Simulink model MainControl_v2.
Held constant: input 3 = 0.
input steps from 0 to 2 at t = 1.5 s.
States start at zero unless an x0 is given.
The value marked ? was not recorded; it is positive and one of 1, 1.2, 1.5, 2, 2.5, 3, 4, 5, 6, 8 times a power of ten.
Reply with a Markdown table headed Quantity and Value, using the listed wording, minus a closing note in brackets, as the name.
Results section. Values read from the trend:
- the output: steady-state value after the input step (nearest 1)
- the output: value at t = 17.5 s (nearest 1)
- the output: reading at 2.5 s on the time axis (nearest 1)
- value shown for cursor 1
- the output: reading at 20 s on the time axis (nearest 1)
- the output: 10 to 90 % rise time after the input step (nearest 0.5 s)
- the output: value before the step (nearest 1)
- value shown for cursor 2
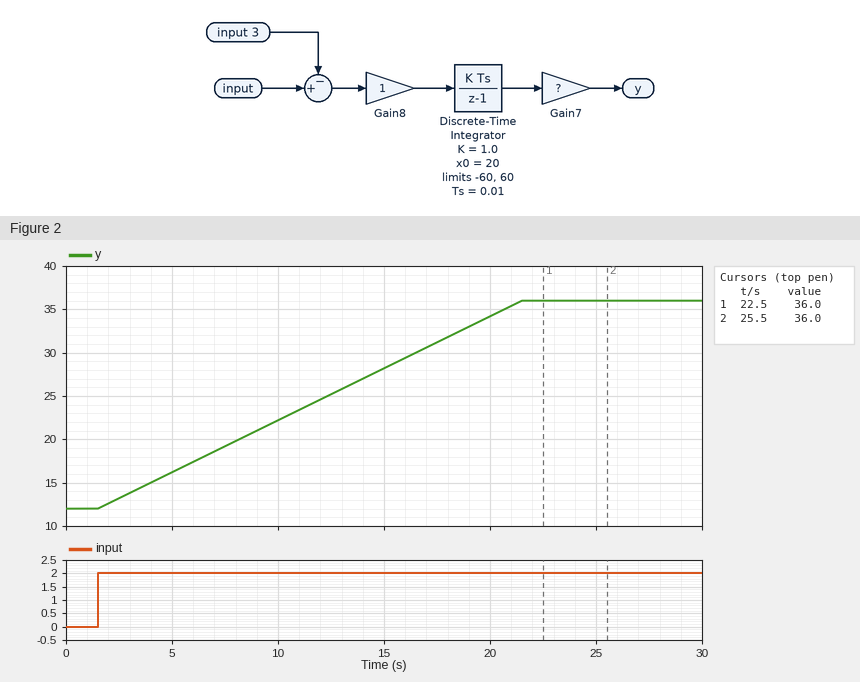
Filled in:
| Quantity | Value |
|---|---|
| the output: steady-state value after the input step | 36 |
| the output: value at t = 17.5 s | 31 |
| the output: reading at 2.5 s on the time axis | 13 |
| value shown for cursor 1 | 36.0 |
| the output: reading at 20 s on the time axis | 34 |
| the output: 10 to 90 % rise time after the input step | 16.0 s |
| the output: value before the step | 12 |
| value shown for cursor 2 | 36.0 |
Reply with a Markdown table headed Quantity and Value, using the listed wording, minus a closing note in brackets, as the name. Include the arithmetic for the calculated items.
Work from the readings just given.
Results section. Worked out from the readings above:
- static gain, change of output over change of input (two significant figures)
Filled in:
| Quantity | Value |
|---|---|
| static gain, change of output over change of input | (36 - 12) / (2 - 0) = 12 |
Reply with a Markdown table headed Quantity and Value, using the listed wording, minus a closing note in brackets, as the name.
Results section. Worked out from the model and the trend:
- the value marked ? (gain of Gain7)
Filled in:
| Quantity | Value |
|---|---|
| the value marked ? | 0.6 |
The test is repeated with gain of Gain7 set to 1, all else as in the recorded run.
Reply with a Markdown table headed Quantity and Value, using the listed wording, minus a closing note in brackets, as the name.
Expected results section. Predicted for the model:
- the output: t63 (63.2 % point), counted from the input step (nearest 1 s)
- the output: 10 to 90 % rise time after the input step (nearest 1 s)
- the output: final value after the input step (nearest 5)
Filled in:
| Quantity | Value |
|---|---|
| the output: t63 (63.2 % point), counted from the input step | 13 s |
| the output: 10 to 90 % rise time after the input step | 16 s |
| the output: final value after the input step | 60 |
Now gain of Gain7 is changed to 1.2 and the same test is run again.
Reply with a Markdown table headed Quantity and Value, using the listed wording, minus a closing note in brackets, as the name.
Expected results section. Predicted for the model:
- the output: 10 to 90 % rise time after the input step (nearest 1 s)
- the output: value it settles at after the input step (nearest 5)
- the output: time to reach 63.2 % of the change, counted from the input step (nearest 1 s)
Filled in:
| Quantity | Value |
|---|---|
| the output: 10 to 90 % rise time after the input step | 16 s |
| the output: value it settles at after the input step | 70 |
| the output: time to reach 63.2 % of the change, counted from the input step | 13 s |
